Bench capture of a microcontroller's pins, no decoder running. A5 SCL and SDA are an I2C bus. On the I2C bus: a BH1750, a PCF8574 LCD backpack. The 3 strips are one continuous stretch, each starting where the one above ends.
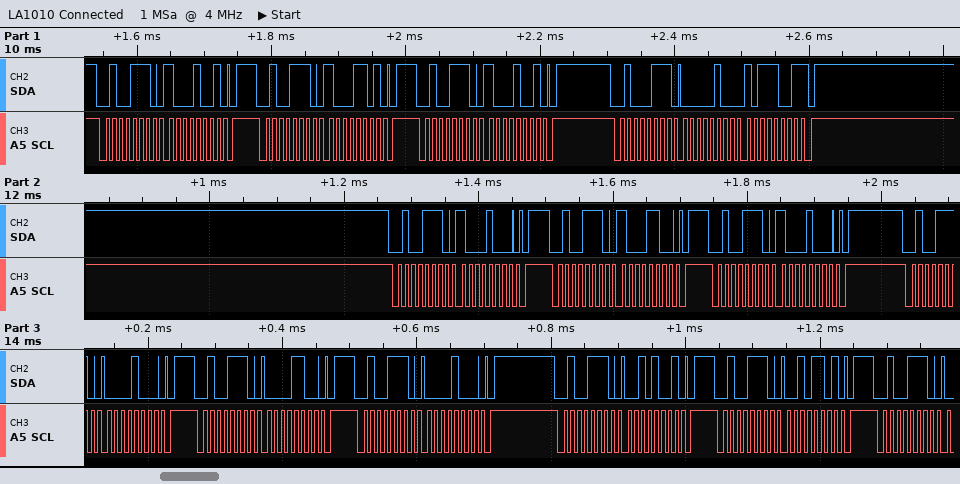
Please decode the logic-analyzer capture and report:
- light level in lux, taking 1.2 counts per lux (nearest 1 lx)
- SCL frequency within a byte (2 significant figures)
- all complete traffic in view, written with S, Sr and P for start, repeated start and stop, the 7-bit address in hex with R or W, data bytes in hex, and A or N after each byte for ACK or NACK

1008 lx
100 kHz
S 27W A 89 A P S 27W A 8D A P S 27W A 89 A P S 23R A 04 A B9 N P S 27W A 88 A P S 27W A 8C A P S 27W A 88 A P S 27W A 08 A P S 27W A 0C A P S 27W A 08 A P S 27W A 29 A P S 27W A 2D A P S 27W A
